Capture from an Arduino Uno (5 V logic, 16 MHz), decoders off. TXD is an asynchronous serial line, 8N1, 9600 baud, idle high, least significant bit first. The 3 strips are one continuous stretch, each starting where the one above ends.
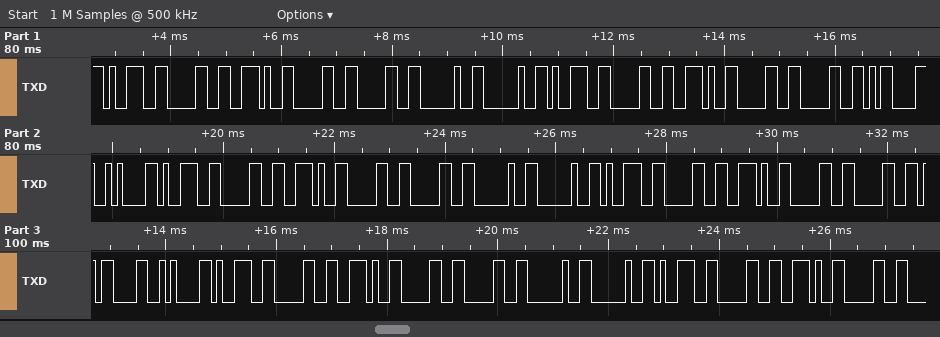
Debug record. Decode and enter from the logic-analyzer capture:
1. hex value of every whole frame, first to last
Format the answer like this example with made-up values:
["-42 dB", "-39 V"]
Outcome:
["39 30 2E 30 30 20 20 39 30 2E 30 30 0D 0A 39 30 2E 30 30 20 20 39 30 2E 30 30 0D 0A 39 30 2E 30 30 20 20 39 30 2E 30"]
